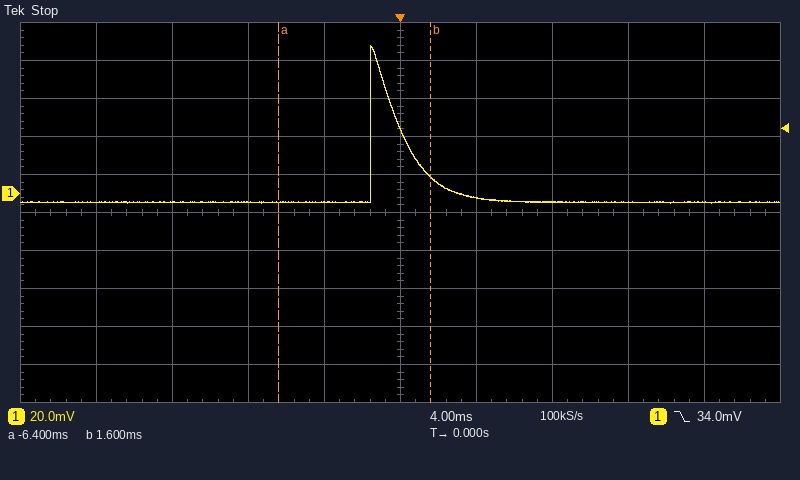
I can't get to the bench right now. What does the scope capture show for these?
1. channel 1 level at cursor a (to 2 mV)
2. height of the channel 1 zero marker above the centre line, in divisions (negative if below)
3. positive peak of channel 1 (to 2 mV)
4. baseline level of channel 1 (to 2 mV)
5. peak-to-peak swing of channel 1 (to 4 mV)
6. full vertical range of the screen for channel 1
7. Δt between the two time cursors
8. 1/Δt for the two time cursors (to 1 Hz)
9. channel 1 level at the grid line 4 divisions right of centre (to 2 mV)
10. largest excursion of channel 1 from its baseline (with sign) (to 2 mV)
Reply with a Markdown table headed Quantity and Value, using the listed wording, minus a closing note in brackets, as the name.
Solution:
| Quantity | Value |
|---|---|
| channel 1 level at cursor a | -4 mV |
| height of the channel 1 zero marker above the centre line, in divisions | +0.5 div |
| positive peak of channel 1 | 78 mV |
| baseline level of channel 1 | -4 mV |
| peak-to-peak swing of channel 1 | 84 mV |
| full vertical range of the screen for channel 1 | 200 mV |
| Δt between the two time cursors | 8.0 ms |
| 1/Δt for the two time cursors | 125 Hz |
| channel 1 level at the grid line 4 divisions right of centre | -4 mV |
| largest excursion of channel 1 from its baseline (with sign) | +82 mV |
